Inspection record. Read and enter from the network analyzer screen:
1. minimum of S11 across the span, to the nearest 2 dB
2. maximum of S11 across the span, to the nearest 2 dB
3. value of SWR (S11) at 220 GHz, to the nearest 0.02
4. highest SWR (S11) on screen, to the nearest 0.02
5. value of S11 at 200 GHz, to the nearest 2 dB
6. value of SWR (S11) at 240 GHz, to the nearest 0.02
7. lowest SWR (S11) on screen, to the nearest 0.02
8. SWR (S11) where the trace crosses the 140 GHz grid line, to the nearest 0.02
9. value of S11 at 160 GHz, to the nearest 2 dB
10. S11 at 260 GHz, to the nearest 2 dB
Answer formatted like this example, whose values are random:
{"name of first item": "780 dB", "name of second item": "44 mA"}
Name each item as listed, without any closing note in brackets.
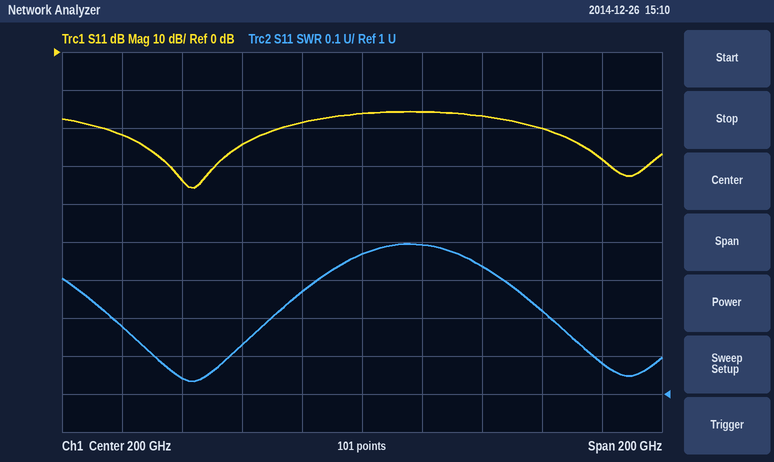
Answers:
{"minimum of S11 across the span, to the nearest 2 dB": "-36 dB", "maximum of S11 across the span, to the nearest 2 dB": "-16 dB", "value of SWR (S11) at 220 GHz, to the nearest 0.02": "1.40", "highest SWR (S11) on screen, to the nearest 0.02": "1.40", "value of S11 at 200 GHz, to the nearest 2 dB": "-16 dB", "value of SWR (S11) at 240 GHz, to the nearest 0.02": "1.34", "lowest SWR (S11) on screen, to the nearest 0.02": "1.04", "SWR (S11) where the trace crosses the 140 GHz grid line, to the nearest 0.02": "1.04", "value of S11 at 160 GHz, to the nearest 2 dB": "-24 dB", "S11 at 260 GHz, to the nearest 2 dB": "-20 dB"}
